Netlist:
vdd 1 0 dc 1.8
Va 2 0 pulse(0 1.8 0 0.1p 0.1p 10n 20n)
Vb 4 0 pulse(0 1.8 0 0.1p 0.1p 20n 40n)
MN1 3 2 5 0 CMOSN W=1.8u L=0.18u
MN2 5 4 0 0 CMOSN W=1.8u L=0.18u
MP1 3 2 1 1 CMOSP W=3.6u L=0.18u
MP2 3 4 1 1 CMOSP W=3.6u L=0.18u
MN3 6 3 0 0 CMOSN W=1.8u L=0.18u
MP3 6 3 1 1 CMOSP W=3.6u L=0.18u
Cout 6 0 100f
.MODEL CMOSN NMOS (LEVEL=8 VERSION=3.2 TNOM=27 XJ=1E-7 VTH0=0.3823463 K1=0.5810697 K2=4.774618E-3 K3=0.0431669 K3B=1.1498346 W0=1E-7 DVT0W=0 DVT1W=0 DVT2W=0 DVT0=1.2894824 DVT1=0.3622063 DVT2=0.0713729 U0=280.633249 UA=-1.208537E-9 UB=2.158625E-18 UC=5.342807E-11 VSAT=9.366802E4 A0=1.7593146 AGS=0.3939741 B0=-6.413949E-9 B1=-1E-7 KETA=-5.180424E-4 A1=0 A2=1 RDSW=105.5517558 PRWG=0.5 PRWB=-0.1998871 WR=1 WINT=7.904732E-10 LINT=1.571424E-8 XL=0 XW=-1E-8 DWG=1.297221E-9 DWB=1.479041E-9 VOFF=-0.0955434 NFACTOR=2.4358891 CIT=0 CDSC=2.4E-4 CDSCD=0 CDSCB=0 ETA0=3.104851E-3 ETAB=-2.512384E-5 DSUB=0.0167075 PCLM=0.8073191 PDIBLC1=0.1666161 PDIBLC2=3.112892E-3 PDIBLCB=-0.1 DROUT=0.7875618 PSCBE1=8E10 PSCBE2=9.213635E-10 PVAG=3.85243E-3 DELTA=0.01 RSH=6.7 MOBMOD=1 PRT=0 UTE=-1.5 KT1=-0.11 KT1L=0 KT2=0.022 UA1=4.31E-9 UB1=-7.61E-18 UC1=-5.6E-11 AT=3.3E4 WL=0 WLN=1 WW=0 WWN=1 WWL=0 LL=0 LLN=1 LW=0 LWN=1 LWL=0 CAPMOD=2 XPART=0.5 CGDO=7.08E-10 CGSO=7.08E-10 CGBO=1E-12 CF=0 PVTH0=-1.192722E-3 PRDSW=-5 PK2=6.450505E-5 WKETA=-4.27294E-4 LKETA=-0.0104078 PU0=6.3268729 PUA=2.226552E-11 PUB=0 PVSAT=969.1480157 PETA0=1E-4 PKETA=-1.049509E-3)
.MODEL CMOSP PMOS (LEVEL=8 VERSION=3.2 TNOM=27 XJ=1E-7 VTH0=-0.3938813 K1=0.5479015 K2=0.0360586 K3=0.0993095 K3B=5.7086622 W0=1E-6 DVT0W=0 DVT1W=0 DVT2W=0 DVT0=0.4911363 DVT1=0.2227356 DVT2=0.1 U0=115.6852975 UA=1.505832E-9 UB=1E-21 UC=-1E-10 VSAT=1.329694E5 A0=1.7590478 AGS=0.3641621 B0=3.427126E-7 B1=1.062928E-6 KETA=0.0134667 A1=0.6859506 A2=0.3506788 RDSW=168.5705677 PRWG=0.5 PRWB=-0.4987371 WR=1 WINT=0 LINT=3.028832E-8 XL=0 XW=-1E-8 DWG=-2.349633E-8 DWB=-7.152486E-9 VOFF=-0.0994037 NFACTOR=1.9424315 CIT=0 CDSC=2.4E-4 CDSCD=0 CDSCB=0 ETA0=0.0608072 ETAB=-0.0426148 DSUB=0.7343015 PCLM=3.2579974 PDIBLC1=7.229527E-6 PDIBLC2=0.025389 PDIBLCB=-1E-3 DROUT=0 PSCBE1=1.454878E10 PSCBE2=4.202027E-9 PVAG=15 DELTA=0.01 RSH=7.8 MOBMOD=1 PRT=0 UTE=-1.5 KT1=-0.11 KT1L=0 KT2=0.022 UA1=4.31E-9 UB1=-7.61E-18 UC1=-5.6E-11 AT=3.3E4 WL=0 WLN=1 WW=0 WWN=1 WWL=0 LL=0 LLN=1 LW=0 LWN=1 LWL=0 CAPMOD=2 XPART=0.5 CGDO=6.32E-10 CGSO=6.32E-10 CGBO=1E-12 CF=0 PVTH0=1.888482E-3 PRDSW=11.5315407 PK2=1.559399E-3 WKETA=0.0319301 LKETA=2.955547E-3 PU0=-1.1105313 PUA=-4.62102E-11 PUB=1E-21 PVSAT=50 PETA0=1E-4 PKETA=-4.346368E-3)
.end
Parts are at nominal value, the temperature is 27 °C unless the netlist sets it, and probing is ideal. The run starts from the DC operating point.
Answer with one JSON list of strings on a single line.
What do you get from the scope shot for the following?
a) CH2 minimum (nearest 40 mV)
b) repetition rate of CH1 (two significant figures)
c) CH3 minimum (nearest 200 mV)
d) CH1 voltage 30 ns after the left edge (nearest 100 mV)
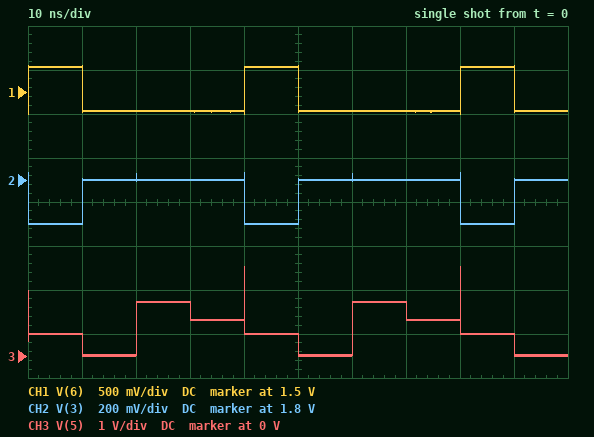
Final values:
["1.60 V", "25 MHz", "0 V", "1.3 V"]
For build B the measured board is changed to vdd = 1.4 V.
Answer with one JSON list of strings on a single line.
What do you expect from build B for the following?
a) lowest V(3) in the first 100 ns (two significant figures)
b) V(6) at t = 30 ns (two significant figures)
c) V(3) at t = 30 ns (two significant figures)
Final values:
["-32 mV", "1.0 V", "1.4 V"]
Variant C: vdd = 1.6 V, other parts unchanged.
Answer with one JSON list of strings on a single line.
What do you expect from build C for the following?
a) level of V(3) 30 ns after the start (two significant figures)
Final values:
["1.6 V"]
